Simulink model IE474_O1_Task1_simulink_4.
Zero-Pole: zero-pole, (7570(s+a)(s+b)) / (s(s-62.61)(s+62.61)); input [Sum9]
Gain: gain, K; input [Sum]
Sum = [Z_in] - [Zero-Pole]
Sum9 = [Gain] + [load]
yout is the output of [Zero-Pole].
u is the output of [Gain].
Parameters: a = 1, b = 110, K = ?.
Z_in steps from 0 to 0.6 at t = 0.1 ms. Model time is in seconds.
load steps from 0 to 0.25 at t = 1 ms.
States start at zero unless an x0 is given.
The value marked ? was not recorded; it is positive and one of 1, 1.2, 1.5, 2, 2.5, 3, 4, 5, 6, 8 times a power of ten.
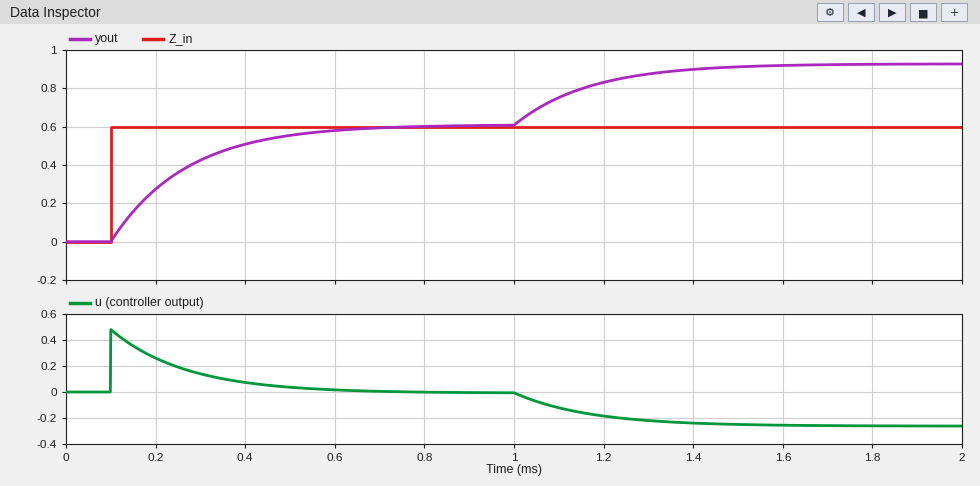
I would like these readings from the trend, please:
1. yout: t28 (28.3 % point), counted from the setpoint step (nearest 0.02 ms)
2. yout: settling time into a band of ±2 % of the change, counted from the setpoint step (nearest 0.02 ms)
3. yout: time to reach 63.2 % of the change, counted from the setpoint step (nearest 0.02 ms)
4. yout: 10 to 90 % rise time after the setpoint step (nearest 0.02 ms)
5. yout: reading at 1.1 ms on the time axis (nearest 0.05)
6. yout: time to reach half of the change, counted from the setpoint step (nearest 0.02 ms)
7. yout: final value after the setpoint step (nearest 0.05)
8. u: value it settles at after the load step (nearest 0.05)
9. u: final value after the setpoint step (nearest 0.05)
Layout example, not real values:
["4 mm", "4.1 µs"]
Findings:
["0.06 ms", "0.60 ms", "0.16 ms", "0.36 ms", "0.75", "0.12 ms", "0.60", "-0.25", "0.00"]
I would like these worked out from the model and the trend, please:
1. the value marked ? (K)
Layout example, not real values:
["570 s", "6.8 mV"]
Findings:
["0.8"]
